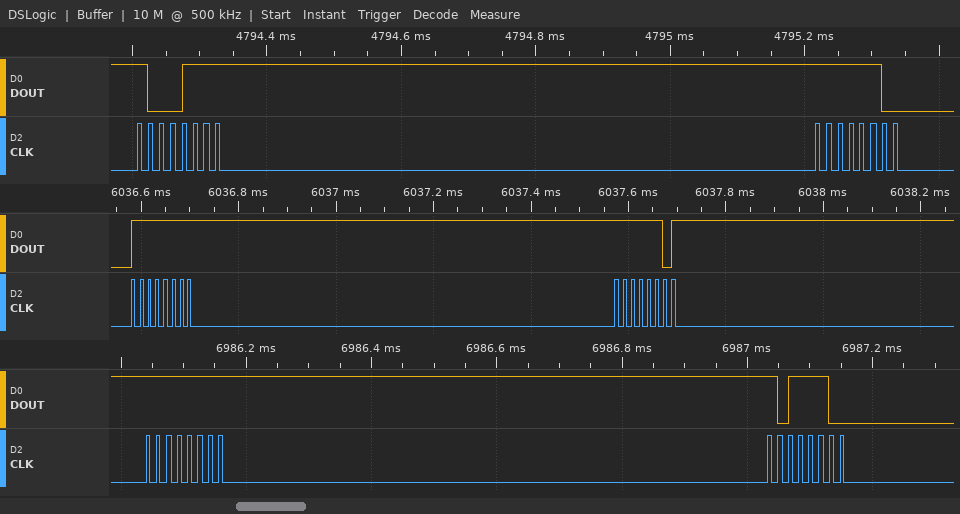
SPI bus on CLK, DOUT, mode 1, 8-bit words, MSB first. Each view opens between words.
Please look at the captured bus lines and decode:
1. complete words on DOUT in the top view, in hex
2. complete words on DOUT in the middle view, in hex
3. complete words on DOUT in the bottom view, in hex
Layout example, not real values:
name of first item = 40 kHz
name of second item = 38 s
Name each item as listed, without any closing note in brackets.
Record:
complete words on DOUT in the top view, in hex = 8F, FC
complete words on DOUT in the middle view, in hex = FF, FD
complete words on DOUT in the bottom view, in hex = FF, BC
